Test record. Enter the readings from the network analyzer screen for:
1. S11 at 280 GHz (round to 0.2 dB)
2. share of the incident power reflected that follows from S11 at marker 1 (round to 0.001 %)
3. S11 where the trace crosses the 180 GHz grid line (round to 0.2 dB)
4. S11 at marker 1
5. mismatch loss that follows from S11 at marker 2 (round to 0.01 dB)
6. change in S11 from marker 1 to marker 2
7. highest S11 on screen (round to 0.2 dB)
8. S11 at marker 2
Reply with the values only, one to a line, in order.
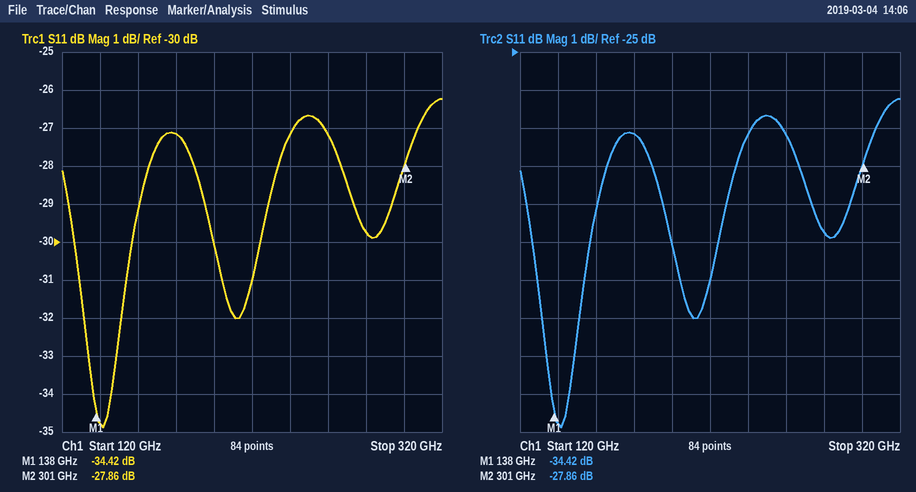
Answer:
-29.8 dB
0.036 %
-27.2 dB
-34.42 dB
0.01 dB
6.56 dB
-26.2 dB
-27.86 dB
